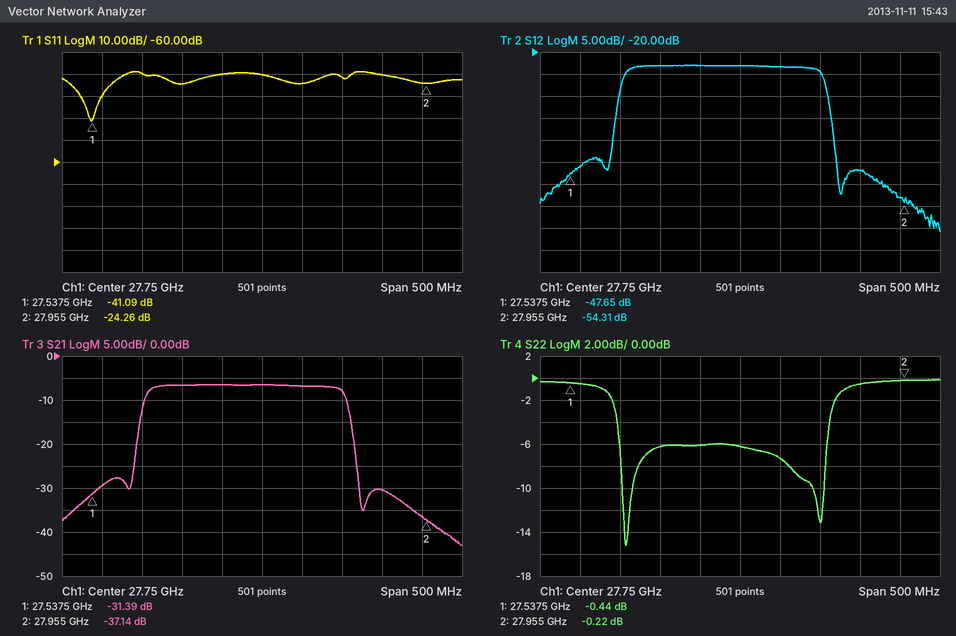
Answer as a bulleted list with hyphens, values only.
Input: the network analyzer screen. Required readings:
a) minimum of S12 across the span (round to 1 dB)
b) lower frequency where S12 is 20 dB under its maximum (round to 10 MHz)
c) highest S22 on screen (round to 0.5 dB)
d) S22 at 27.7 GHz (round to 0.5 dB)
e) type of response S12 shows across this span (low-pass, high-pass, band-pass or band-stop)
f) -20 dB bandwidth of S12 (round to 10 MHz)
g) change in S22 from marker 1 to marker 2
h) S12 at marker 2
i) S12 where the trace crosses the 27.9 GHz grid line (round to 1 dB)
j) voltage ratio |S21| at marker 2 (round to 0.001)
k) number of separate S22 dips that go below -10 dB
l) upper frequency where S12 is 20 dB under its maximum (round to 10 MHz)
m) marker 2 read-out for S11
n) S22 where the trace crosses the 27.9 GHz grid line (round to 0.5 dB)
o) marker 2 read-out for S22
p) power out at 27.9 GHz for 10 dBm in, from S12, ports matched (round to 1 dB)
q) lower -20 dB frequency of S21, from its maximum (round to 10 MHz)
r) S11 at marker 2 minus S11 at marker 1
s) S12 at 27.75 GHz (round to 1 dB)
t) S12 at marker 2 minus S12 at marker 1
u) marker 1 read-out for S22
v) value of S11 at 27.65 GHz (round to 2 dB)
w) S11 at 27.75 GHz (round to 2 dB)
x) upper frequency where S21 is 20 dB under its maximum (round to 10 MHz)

- -61 dB
- 27.59 GHz
- 0.0 dB
- -6.0 dB
- band-pass
- 280 MHz
- 0.22 dB
- -54.31 dB
- -47 dB
- 0.014
- 2
- 27.87 GHz
- -24.26 dB
- -0.5 dB
- -0.22 dB
- -37 dBm
- 27.59 GHz
- 16.83 dB
- -23 dB
- -6.66 dB
- -0.44 dB
- -24 dB
- -20 dB
- 27.87 GHz
